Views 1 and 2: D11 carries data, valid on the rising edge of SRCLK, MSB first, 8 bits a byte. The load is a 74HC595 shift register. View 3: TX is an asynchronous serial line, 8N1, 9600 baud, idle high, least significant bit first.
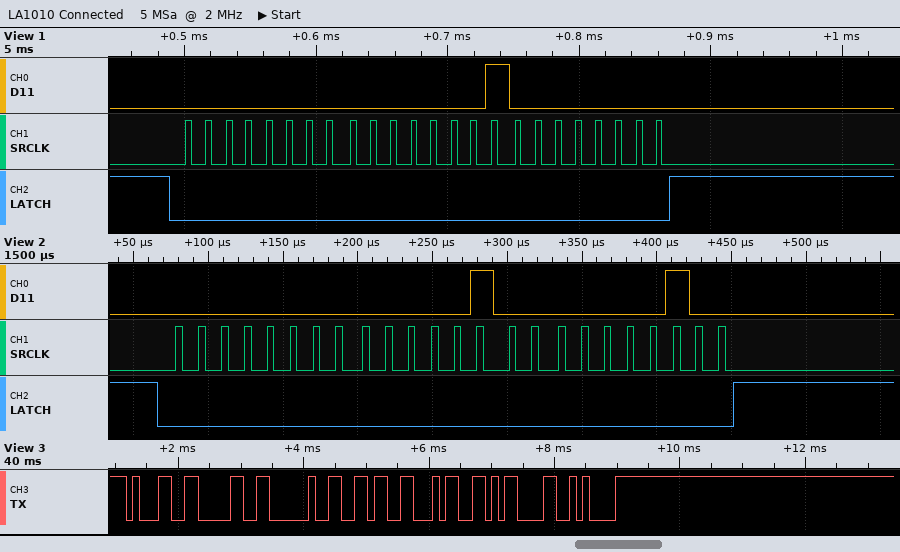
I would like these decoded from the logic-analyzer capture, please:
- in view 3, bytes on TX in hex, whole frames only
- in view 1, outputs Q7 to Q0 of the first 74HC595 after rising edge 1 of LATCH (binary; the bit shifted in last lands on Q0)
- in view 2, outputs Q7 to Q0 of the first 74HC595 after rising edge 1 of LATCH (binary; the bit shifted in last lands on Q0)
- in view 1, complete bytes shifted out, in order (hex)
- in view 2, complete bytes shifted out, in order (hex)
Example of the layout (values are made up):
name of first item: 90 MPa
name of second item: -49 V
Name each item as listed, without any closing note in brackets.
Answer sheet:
in view 3, bytes on TX in hex, whole frames only: 31 30 20 36 34 0D 0A
in view 1, outputs Q7 to Q0 of the first 74HC595 after rising edge 1 of LATCH: 00000000
in view 2, outputs Q7 to Q0 of the first 74HC595 after rising edge 1 of LATCH: 00000100
in view 1, complete bytes shifted out, in order: 00 01 00
in view 2, complete bytes shifted out, in order: 00 04 04
